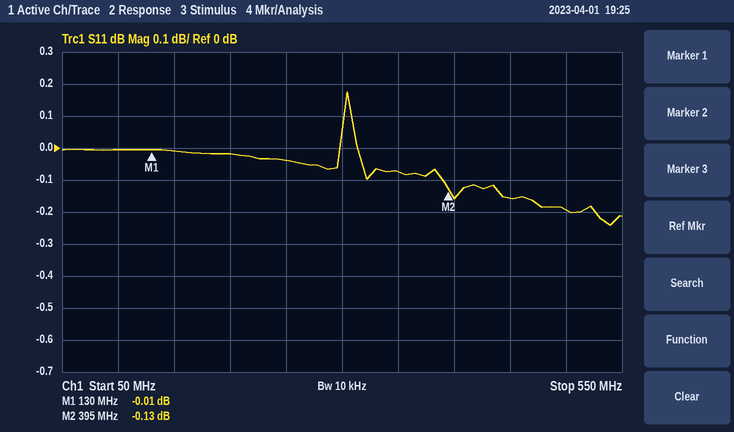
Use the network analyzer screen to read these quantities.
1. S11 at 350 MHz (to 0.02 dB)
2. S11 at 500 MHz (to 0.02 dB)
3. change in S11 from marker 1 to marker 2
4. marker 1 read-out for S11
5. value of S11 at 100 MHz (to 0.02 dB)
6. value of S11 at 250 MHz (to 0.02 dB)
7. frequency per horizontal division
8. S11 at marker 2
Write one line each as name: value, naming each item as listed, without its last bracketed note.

S11 at 350 MHz: -0.08 dB
S11 at 500 MHz: -0.20 dB
change in S11 from marker 1 to marker 2: -0.12 dB
marker 1 read-out for S11: -0.01 dB
value of S11 at 100 MHz: 0.00 dB
value of S11 at 250 MHz: -0.04 dB
frequency per horizontal division: 50 MHz
S11 at marker 2: -0.13 dB
